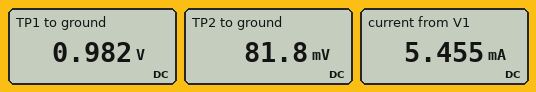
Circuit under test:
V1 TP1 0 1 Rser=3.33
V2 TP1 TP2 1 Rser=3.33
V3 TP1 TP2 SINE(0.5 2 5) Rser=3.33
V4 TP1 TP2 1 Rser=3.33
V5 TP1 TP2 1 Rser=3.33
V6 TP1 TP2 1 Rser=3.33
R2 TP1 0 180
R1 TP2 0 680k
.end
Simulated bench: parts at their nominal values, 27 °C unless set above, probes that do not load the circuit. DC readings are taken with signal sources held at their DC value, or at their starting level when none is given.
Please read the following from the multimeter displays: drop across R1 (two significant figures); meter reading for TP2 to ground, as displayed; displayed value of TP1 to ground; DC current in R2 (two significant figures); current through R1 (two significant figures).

82 mV
81.8 mV
0.982 V
5.5 mA
120 nA
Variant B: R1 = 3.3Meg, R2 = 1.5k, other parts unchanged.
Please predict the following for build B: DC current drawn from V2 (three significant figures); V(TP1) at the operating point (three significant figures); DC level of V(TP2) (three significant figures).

30.0 mA
998 mV
97.8 mV
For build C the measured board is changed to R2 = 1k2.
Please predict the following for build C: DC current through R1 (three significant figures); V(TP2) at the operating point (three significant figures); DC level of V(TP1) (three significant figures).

143 nA
97.2 mV
997 mV
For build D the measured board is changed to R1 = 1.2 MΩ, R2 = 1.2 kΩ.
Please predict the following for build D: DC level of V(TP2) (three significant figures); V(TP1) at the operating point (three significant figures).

97.2 mV
997 mV
